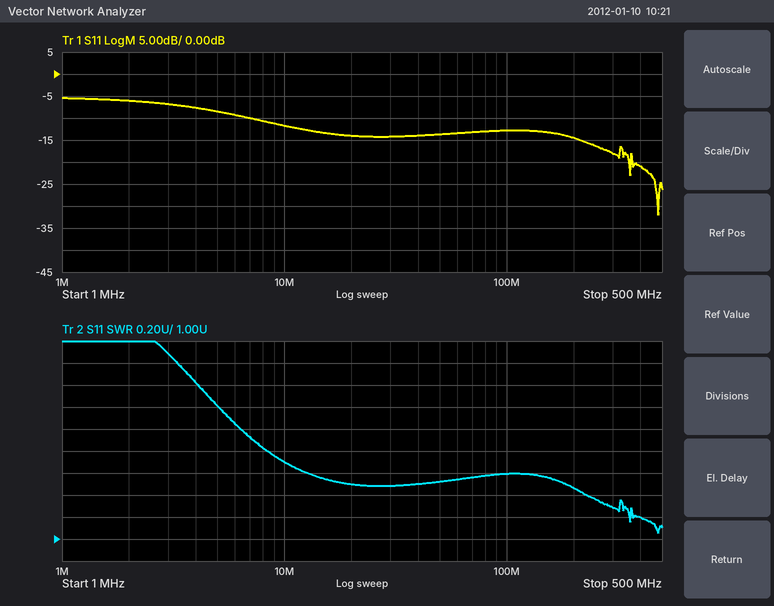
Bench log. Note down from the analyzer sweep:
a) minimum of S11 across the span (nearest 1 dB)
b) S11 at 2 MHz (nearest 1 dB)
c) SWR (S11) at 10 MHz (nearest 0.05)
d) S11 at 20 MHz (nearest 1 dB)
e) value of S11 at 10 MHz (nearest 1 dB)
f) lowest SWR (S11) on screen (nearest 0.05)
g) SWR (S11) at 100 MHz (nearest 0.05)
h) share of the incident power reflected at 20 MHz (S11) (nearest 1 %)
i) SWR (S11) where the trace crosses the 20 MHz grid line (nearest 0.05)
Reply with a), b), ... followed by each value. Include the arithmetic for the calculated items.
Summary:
a) -32 dB
b) -6 dB
c) 1.70
d) -14 dB
e) -12 dB
f) 1.05
g) 1.60
h) 10^(-14/10) ≈ 4 %
i) 1.50
